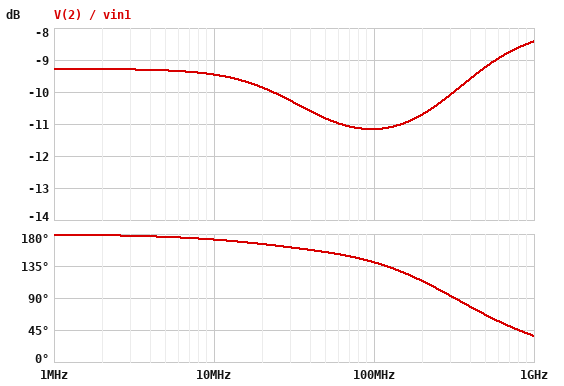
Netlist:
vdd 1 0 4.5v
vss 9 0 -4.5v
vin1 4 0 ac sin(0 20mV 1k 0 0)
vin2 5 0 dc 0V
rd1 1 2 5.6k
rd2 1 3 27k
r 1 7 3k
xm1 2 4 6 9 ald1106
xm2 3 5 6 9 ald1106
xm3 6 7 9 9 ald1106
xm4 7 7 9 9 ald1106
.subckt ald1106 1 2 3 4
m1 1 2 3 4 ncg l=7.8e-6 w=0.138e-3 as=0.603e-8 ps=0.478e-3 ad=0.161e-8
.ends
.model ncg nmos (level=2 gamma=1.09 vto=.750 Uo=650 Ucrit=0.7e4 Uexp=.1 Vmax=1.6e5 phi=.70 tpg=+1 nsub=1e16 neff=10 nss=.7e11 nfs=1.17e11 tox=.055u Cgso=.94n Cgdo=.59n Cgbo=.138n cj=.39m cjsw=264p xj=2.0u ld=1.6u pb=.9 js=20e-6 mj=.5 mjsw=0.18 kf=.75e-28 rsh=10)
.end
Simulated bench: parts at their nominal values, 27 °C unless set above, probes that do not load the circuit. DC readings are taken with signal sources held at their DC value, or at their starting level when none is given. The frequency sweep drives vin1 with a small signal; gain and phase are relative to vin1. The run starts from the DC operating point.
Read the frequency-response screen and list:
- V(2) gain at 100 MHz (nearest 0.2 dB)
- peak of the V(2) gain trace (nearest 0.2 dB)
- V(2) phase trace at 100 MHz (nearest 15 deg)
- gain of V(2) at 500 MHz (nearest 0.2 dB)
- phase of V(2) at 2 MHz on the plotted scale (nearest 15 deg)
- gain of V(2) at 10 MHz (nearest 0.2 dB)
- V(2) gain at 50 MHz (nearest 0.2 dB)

-11.2 dB
-8.4 dB
135 deg
-9.2 dB
180 deg
-9.4 dB
-10.8 dB
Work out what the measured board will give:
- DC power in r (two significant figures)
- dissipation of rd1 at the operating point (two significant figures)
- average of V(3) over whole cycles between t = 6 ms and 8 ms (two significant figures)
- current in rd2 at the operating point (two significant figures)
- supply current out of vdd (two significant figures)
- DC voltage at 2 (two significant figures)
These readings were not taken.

11 mW
9.1 mW
-3.3 V
290 µA
3.5 mA
-2.6 V
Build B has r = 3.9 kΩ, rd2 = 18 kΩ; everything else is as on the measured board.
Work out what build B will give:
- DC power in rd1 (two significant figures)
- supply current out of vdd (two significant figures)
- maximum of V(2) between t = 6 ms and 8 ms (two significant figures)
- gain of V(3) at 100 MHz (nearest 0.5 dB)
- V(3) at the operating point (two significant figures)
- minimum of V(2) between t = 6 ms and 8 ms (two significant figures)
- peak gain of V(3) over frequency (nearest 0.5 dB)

6.8 mW
3.1 mA
-1.6 V
-10.0 dB
-2.7 V
-1.7 V
-3.0 dB
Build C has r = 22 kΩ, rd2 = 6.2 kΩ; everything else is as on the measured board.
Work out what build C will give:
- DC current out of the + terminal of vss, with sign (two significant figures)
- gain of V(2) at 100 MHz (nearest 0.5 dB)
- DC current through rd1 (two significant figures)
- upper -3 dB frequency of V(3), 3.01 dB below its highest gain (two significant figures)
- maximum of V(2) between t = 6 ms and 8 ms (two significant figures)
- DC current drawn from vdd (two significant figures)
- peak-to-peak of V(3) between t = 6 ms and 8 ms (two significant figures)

-670 µA
4.0 dB
170 µA
43 MHz
3.6 V
670 µA
61 mV
